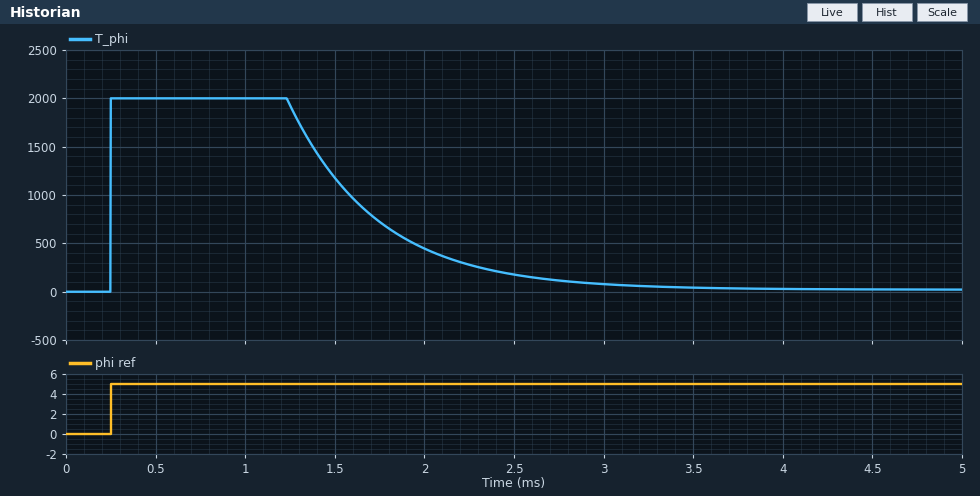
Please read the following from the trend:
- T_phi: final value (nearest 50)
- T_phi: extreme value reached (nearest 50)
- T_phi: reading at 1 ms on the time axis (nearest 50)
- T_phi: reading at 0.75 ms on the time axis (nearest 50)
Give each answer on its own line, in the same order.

0
2000
2000
2000
